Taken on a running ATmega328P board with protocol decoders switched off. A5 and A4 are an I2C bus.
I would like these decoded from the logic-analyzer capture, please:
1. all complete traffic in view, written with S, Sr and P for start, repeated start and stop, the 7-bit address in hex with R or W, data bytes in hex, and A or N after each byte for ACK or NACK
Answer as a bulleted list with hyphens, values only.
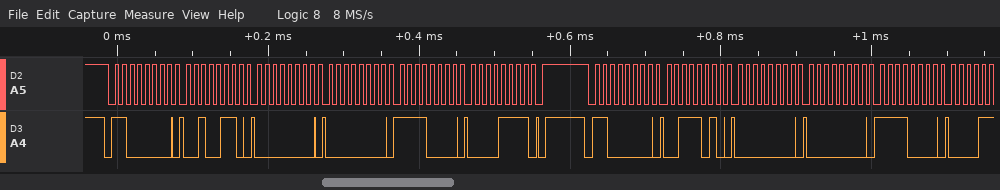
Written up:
- S 60W A 26 A 00 A 00 A F0 A 0F A P S 60W A 3A A 00 A 00 A F0 A
